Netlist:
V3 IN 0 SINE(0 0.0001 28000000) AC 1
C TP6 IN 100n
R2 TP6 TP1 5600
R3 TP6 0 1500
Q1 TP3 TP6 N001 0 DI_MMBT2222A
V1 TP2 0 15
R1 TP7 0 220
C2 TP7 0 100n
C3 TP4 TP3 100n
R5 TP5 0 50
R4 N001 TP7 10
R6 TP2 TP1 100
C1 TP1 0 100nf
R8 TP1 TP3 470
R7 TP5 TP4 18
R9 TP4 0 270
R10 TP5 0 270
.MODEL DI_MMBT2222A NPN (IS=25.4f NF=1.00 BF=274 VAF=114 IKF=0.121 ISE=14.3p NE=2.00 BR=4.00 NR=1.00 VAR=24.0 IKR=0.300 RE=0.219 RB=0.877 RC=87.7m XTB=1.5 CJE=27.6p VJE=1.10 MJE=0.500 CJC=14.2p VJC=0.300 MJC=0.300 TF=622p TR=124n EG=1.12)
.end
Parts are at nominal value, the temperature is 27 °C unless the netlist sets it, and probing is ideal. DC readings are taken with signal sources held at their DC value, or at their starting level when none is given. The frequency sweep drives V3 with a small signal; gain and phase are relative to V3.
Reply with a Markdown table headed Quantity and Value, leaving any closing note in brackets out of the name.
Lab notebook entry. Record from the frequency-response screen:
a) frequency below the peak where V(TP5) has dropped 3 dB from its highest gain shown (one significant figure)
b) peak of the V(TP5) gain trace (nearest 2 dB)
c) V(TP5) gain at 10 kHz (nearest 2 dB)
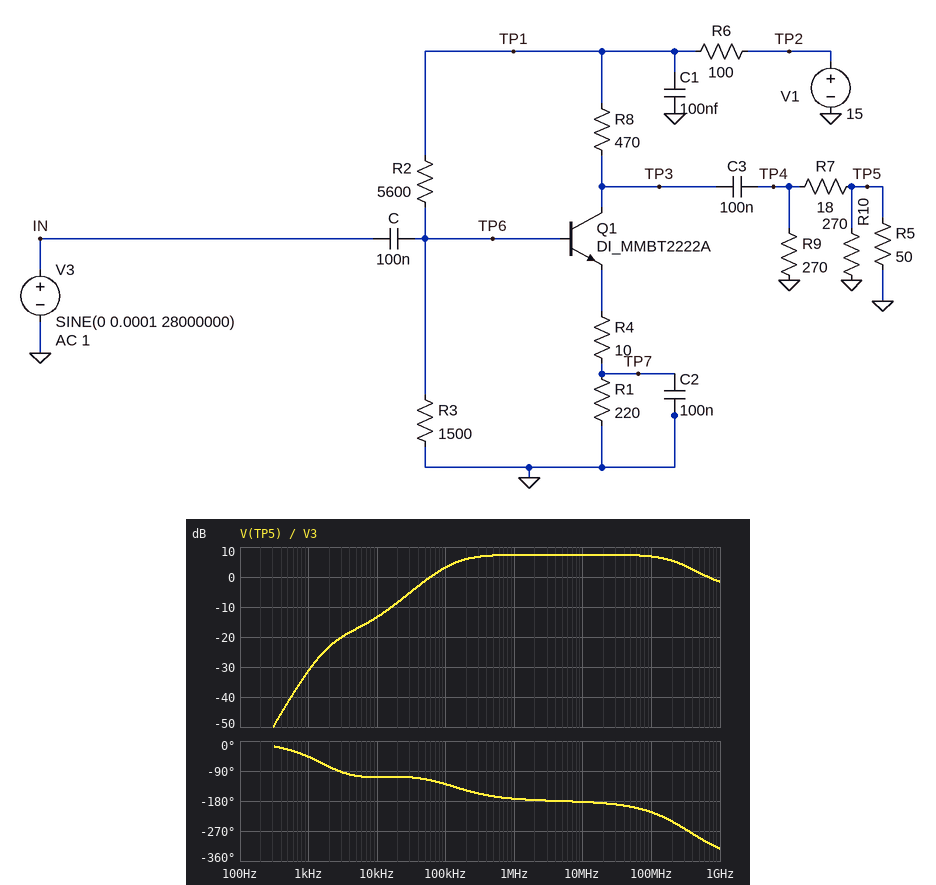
| Quantity | Value |
|---|---|
| frequency below the peak where V(TP5) has dropped 3 dB from its highest gain shown | 100 kHz |
| peak of the V(TP5) gain trace | 8 dB |
| V(TP5) gain at 10 kHz | -14 dB |
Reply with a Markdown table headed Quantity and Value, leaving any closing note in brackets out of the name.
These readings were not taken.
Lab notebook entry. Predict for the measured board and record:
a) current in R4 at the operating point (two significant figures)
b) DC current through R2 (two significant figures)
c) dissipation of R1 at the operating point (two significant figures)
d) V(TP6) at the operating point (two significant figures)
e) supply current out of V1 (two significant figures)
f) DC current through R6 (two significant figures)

| Quantity | Value |
|---|---|
| current in R4 at the operating point | 9.5 mA |
| DC current through R2 | 2.0 mA |
| dissipation of R1 at the operating point | 20 mW |
| V(TP6) at the operating point | 2.9 V |
| supply current out of V1 | 11 mA |
| DC current through R6 | 11 mA |
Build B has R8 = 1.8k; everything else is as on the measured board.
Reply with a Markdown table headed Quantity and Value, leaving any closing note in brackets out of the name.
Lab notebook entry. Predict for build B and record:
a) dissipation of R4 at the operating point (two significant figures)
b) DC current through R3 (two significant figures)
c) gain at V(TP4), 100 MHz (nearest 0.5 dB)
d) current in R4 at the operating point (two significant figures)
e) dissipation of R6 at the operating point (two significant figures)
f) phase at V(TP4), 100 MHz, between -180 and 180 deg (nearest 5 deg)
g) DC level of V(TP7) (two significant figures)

| Quantity | Value |
|---|---|
| dissipation of R4 at the operating point | 540 µW |
| DC current through R3 | 1.6 mA |
| gain at V(TP4), 100 MHz | -0.5 dB |
| current in R4 at the operating point | 7.4 mA |
| dissipation of R6 at the operating point | 8.0 mW |
| phase at V(TP4), 100 MHz, between -180 and 180 deg | 0 deg |
| DC level of V(TP7) | 1.6 V |
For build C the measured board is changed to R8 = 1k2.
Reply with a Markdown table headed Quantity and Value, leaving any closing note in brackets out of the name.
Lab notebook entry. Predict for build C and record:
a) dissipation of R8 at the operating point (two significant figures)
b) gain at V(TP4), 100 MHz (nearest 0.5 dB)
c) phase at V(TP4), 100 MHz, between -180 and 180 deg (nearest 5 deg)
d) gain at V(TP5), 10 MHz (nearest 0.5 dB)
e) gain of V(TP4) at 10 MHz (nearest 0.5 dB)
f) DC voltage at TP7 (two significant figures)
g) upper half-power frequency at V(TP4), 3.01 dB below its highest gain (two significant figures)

| Quantity | Value |
|---|---|
| dissipation of R8 at the operating point | 110 mW |
| gain at V(TP4), 100 MHz | 9.0 dB |
| phase at V(TP4), 100 MHz, between -180 and 180 deg | 110 deg |
| gain at V(TP5), 10 MHz | 8.0 dB |
| gain of V(TP4) at 10 MHz | 11.0 dB |
| DC voltage at TP7 | 2.1 V |
| upper half-power frequency at V(TP4), 3.01 dB below its highest gain | 140 MHz |
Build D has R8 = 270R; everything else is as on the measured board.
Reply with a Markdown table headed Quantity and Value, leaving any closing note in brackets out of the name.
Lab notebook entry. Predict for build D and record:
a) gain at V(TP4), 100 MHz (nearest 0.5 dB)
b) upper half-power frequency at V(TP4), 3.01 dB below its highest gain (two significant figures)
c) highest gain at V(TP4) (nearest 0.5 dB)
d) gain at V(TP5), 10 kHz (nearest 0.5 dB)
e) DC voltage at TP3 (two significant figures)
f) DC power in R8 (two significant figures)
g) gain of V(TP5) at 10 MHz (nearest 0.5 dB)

| Quantity | Value |
|---|---|
| gain at V(TP4), 100 MHz | 9.5 dB |
| upper half-power frequency at V(TP4), 3.01 dB below its highest gain | 270 MHz |
| highest gain at V(TP4) | 10.0 dB |
| gain at V(TP5), 10 kHz | -14.5 dB |
| DC voltage at TP3 | 11 V |
| DC power in R8 | 24 mW |
| gain of V(TP5) at 10 MHz | 7.0 dB |
